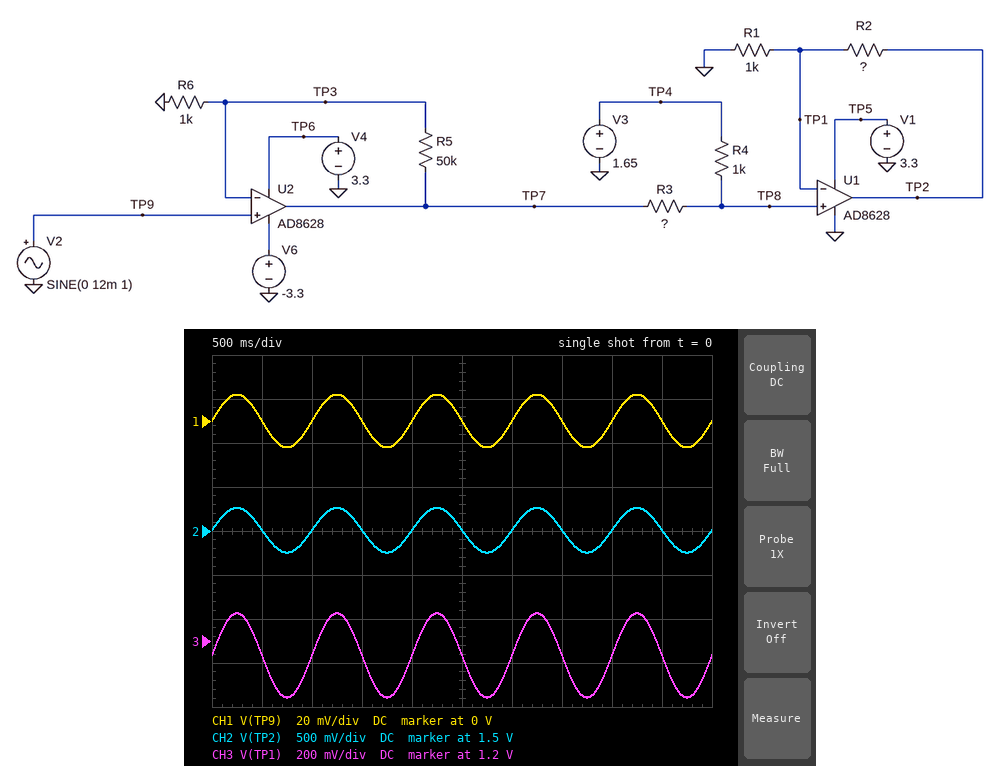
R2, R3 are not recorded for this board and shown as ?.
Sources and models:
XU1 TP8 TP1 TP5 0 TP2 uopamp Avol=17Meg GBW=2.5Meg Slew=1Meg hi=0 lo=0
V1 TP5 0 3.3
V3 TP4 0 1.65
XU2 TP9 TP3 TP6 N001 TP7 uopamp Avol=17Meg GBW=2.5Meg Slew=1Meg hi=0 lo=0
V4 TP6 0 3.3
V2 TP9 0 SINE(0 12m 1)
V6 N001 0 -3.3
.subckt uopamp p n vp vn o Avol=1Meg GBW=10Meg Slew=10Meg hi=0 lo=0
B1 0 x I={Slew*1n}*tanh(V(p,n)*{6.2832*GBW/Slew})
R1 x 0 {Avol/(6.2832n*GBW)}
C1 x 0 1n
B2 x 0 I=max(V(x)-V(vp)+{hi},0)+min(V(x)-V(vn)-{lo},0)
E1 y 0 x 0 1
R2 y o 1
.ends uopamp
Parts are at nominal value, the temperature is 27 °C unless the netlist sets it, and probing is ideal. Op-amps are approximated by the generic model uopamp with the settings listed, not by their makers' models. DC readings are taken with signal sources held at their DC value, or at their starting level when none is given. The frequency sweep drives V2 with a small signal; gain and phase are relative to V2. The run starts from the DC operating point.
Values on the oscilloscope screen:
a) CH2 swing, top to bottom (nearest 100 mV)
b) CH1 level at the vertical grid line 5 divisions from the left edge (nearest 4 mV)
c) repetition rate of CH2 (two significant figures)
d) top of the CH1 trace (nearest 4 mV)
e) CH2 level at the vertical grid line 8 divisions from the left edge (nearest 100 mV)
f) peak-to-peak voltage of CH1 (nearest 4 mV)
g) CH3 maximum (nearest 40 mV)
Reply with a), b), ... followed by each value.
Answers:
a) 500 mV
b) 0 V
c) 1.0 Hz
d) 12 mV
e) 1.5 V
f) 24 mV
g) 1.32 V
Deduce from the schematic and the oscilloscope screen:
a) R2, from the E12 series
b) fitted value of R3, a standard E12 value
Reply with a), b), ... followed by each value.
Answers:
a) 330 Ω
b) 2.2 kΩ
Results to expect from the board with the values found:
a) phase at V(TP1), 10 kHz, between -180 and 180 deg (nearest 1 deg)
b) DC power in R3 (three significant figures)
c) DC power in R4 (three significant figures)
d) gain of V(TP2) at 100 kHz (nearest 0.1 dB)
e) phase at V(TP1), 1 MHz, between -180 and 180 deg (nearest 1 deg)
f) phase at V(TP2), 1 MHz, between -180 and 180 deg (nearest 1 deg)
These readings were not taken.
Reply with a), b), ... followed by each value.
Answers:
a) -12 deg
b) 585 µW
c) 266 µW
d) 19.4 dB
e) -115 deg
f) -115 deg
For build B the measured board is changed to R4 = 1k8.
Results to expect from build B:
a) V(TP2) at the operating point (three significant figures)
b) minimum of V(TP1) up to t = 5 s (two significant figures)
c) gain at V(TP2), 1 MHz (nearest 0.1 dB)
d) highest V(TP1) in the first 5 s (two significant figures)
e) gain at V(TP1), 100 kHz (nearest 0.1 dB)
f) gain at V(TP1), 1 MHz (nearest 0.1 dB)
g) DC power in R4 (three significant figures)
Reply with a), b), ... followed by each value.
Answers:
a) 1.21 V
b) 630 mV
c) 2.4 dB
d) 1.2 V
e) 20.1 dB
f) -0.1 dB
g) 306 µW
